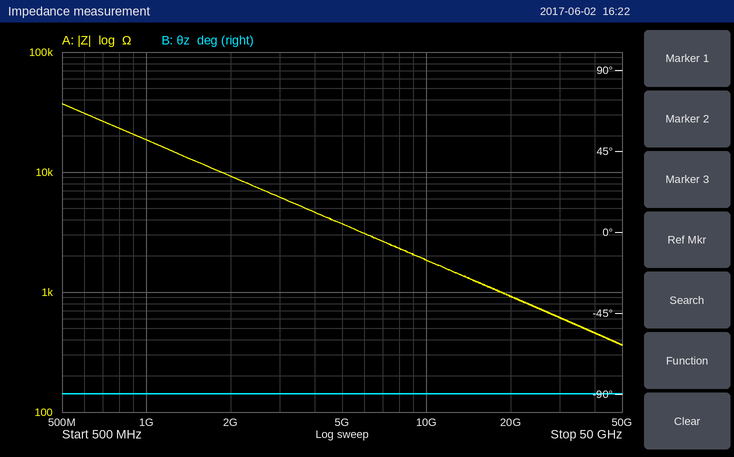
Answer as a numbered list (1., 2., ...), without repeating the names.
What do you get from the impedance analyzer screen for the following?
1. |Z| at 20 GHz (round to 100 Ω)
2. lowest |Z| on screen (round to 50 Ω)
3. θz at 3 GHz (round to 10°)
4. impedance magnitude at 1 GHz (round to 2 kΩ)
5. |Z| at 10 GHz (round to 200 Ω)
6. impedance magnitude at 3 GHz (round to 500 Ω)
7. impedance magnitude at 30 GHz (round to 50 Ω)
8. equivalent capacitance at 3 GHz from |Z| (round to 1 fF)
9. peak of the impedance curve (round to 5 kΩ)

1. 900 Ω
2. 350 Ω
3. -90°
4. 18 kΩ
5. 1.8 kΩ
6. 6.0 kΩ
7. 600 Ω
8. 9 fF
9. 35 kΩ
